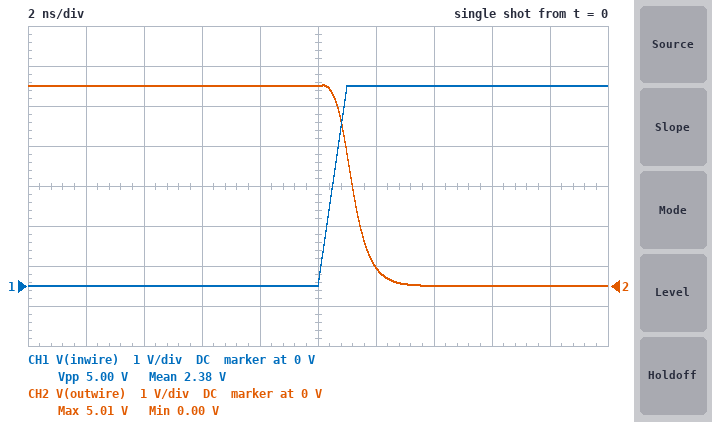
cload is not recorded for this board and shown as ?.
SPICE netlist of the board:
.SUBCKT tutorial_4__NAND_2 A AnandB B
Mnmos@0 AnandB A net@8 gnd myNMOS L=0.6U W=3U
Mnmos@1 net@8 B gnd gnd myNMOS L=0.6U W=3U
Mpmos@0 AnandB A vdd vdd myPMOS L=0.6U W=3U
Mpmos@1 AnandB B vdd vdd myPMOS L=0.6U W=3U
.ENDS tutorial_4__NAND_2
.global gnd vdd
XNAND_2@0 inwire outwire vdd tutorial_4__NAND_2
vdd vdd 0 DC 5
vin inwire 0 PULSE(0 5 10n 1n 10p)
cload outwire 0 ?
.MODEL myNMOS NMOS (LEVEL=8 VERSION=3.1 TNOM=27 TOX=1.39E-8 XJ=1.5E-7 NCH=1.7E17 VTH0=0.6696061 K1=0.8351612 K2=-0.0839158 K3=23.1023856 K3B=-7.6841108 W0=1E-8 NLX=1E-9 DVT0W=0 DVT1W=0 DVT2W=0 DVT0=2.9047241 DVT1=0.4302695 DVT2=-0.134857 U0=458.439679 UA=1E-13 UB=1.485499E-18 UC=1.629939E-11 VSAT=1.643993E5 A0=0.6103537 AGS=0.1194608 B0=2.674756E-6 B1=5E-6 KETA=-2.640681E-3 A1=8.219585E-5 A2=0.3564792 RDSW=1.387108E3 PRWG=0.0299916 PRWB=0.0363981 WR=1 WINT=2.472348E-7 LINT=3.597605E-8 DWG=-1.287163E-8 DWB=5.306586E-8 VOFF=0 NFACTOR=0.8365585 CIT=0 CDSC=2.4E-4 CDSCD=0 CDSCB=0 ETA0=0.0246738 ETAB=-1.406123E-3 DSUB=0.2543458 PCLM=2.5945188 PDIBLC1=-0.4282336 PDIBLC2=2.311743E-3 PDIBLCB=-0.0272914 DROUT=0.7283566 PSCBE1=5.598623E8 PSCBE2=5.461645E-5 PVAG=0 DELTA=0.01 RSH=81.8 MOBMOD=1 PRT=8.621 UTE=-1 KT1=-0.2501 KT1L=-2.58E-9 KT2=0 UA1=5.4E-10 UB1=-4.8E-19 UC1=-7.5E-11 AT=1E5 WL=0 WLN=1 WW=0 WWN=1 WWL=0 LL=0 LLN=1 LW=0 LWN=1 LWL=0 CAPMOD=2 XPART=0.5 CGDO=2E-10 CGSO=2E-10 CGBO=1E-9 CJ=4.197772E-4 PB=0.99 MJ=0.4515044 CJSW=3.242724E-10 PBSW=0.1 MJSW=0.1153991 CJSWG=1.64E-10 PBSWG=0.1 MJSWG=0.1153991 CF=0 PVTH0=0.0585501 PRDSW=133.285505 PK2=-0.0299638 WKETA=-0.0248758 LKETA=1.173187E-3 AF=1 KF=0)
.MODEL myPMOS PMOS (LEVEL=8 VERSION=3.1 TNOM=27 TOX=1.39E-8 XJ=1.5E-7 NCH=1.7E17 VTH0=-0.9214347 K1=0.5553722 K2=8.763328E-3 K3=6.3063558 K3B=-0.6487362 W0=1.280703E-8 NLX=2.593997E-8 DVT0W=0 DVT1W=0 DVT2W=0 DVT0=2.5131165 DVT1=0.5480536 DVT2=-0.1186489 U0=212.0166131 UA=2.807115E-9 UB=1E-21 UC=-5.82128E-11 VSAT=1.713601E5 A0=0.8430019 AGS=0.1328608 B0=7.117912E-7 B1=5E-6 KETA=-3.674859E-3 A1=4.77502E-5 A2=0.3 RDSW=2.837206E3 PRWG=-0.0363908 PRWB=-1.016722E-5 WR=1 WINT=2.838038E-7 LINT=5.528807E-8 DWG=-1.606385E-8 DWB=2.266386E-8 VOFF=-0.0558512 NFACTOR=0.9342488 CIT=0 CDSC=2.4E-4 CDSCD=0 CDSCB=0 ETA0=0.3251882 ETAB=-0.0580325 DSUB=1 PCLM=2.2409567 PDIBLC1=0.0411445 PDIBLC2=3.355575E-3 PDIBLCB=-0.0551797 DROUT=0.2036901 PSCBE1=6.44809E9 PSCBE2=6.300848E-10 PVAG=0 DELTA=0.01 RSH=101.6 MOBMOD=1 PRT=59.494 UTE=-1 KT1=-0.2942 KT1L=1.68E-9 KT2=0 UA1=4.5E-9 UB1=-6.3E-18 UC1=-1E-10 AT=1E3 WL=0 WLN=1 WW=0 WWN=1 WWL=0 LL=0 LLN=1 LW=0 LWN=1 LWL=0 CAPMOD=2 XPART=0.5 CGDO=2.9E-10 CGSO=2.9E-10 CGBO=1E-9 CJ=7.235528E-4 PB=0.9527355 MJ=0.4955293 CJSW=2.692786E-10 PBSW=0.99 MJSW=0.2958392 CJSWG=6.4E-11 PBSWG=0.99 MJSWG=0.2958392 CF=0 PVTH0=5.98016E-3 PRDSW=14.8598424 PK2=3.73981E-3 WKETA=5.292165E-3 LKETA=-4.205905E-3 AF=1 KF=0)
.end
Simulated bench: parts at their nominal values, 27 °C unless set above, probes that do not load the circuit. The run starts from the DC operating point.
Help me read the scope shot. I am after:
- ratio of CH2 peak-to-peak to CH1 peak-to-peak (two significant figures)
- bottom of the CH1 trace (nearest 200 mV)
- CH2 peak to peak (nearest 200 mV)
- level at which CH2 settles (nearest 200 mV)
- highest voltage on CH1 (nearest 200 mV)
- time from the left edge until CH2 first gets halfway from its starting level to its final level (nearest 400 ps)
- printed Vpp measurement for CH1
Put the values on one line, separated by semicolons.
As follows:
1.0; 0 V; 5.0 V; 0 V; 5.0 V; 11.2 ns; 5.00 V
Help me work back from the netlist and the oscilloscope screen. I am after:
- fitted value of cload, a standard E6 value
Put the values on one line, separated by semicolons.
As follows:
150 fF
